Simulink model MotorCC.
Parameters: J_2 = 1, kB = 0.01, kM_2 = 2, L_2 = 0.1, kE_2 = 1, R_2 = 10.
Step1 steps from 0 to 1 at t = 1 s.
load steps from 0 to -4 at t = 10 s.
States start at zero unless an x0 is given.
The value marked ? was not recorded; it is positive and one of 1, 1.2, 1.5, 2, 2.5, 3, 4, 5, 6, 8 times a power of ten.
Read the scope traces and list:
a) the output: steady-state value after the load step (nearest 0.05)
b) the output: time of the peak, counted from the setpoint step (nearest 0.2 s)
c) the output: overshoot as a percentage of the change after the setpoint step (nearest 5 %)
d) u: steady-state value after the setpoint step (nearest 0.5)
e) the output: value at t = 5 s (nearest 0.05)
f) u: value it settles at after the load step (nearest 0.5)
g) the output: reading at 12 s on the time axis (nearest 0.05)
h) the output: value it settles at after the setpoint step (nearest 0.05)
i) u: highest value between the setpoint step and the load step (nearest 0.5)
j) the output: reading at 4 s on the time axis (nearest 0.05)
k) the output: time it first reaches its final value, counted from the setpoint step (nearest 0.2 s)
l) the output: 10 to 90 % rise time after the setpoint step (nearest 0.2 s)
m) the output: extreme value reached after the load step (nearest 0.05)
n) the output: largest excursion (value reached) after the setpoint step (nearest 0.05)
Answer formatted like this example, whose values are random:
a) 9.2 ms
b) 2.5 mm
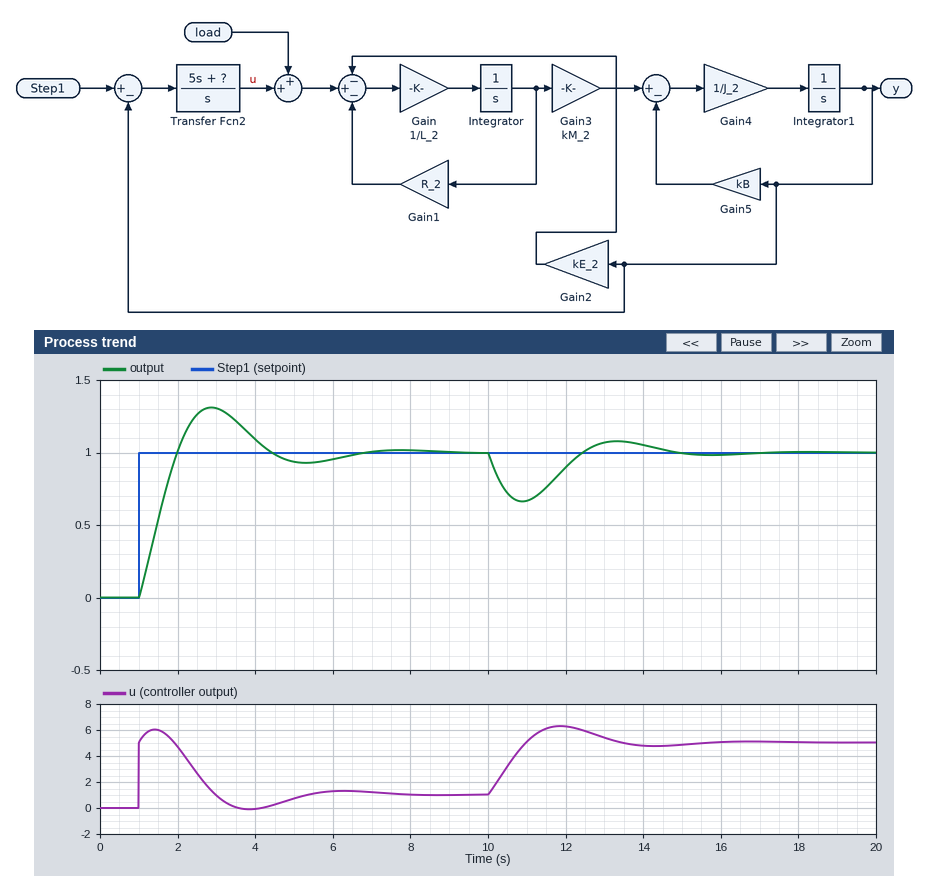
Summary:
a) 1.00
b) 1.8 s
c) 30 %
d) 1.0
e) 0.95
f) 5.0
g) 0.90
h) 1.00
i) 6.0
j) 1.10
k) 1.0 s
l) 0.8 s
m) 0.65
n) 1.30
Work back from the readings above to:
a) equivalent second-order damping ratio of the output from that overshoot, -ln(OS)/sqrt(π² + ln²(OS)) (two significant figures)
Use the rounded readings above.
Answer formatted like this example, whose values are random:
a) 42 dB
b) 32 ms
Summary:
a) 0.36
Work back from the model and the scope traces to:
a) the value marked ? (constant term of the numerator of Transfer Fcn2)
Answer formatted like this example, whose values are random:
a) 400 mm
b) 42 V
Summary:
a) 10
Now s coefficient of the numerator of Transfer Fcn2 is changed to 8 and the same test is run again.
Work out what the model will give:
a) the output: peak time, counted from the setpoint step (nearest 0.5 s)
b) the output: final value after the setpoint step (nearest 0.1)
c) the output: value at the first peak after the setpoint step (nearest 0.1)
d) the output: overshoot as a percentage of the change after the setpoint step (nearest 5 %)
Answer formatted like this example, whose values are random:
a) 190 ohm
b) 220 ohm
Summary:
a) 1.5 s
b) 1.0
c) 1.2
d) 20 %
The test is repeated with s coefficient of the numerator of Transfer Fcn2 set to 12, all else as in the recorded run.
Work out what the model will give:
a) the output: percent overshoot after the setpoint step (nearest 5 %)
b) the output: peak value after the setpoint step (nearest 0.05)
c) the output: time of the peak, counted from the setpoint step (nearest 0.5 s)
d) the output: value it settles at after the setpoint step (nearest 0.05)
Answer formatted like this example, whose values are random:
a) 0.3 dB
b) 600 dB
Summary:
a) 10 %
b) 1.10
c) 1.5 s
d) 1.00
